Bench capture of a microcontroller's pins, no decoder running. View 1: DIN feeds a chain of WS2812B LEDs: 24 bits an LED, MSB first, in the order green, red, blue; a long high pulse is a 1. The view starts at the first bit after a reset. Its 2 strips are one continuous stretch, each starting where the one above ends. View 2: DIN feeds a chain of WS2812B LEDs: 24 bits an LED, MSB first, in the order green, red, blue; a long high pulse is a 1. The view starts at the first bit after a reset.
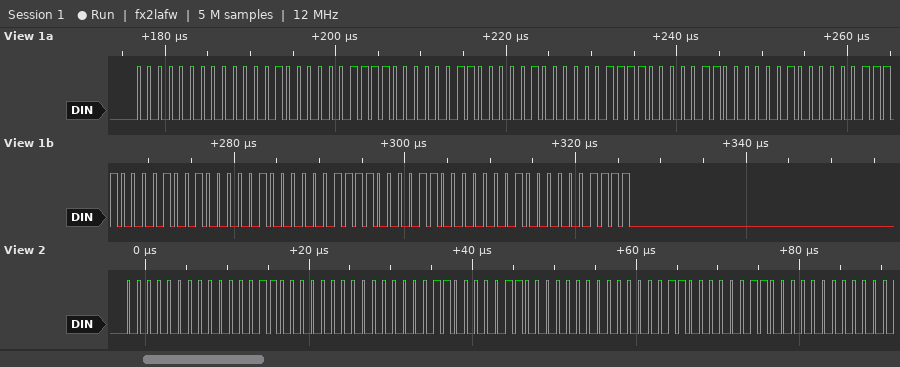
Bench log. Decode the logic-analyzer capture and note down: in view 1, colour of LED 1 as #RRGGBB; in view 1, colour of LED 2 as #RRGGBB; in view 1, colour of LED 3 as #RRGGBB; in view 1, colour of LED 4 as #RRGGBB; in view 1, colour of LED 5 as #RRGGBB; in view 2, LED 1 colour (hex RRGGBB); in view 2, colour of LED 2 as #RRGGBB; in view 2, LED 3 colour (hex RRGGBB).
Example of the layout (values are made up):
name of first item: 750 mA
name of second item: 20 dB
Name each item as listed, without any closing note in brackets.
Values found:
in view 1, colour of LED 1 as #RRGGBB: #04000F
in view 1, colour of LED 2 as #RRGGBB: #04030F
in view 1, colour of LED 3 as #RRGGBB: #04060F
in view 1, colour of LED 4 as #RRGGBB: #04090F
in view 1, colour of LED 5 as #RRGGBB: #040C0F
in view 2, LED 1 colour: #060000
in view 2, colour of LED 2 as #RRGGBB: #060300
in view 2, LED 3 colour: #060600
